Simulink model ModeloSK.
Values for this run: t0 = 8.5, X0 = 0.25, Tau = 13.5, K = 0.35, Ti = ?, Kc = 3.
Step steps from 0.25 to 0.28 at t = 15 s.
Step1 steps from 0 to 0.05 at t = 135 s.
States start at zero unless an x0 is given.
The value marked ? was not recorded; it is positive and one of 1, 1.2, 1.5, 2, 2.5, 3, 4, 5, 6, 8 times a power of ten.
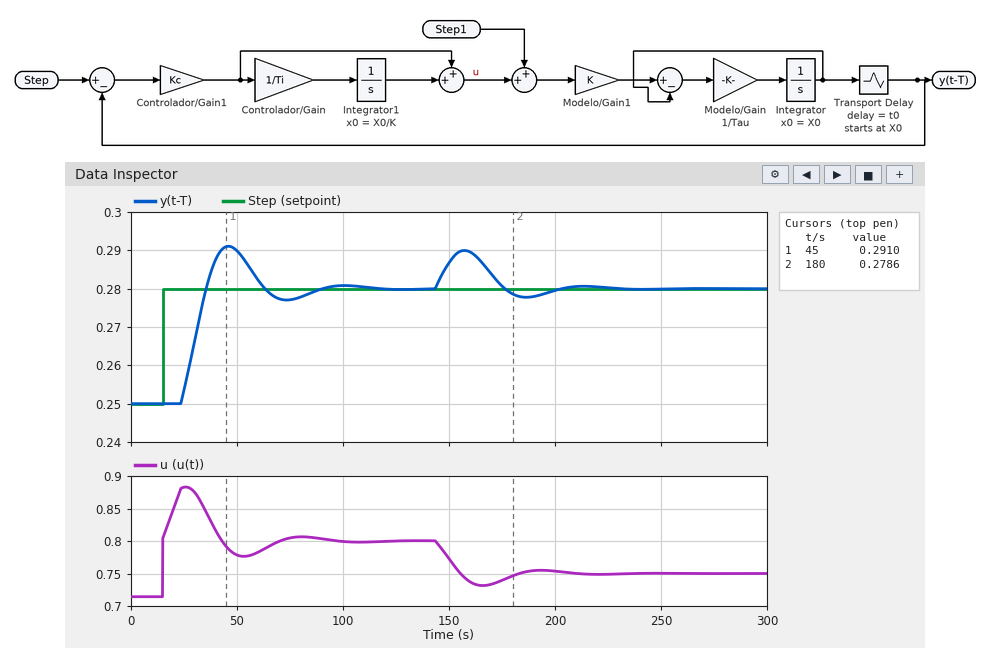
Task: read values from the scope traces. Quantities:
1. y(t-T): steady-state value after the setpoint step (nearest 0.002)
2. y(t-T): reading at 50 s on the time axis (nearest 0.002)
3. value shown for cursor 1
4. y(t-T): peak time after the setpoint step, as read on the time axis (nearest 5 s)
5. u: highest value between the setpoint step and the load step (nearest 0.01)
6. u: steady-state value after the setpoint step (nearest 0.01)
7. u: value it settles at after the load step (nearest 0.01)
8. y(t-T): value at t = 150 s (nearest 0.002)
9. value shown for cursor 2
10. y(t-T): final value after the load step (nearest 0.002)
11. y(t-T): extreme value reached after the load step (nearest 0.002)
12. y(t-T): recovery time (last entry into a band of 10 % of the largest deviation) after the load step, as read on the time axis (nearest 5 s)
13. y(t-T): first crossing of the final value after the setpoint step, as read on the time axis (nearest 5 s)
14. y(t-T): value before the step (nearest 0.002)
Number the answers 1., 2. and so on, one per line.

1. 0.280
2. 0.290
3. 0.2910
4. 45 s
5. 0.88
6. 0.80
7. 0.75
8. 0.286
9. 0.2786
10. 0.280
11. 0.290
12. 195 s
13. 35 s
14. 0.250
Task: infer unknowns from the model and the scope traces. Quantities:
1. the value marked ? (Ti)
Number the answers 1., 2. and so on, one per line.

1. 10
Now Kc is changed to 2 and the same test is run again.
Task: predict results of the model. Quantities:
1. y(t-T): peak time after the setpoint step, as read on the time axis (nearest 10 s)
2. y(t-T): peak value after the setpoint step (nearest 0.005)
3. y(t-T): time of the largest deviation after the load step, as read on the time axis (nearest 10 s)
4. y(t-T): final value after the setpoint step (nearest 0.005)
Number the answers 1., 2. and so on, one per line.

1. 60 s
2. 0.285
3. 160 s
4. 0.280
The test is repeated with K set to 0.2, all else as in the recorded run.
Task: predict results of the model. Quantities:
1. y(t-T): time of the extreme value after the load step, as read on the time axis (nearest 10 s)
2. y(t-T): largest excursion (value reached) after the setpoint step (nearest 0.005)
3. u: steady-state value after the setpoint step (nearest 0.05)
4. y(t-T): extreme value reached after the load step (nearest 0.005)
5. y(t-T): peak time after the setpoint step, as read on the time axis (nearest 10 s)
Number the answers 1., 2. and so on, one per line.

1. 160 s
2. 0.285
3. 1.40
4. 0.285
5. 60 s
